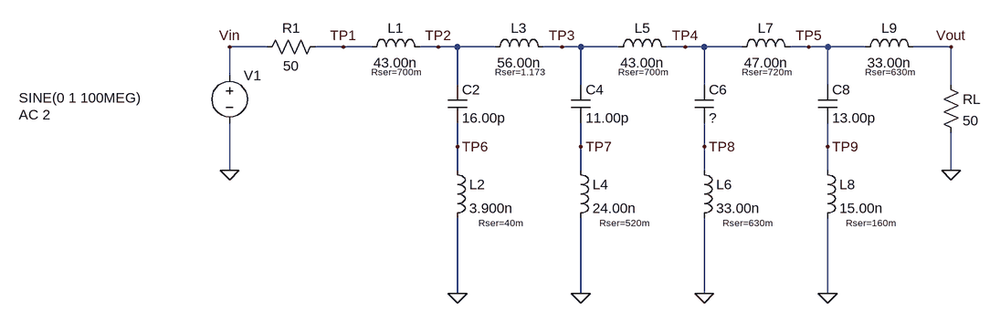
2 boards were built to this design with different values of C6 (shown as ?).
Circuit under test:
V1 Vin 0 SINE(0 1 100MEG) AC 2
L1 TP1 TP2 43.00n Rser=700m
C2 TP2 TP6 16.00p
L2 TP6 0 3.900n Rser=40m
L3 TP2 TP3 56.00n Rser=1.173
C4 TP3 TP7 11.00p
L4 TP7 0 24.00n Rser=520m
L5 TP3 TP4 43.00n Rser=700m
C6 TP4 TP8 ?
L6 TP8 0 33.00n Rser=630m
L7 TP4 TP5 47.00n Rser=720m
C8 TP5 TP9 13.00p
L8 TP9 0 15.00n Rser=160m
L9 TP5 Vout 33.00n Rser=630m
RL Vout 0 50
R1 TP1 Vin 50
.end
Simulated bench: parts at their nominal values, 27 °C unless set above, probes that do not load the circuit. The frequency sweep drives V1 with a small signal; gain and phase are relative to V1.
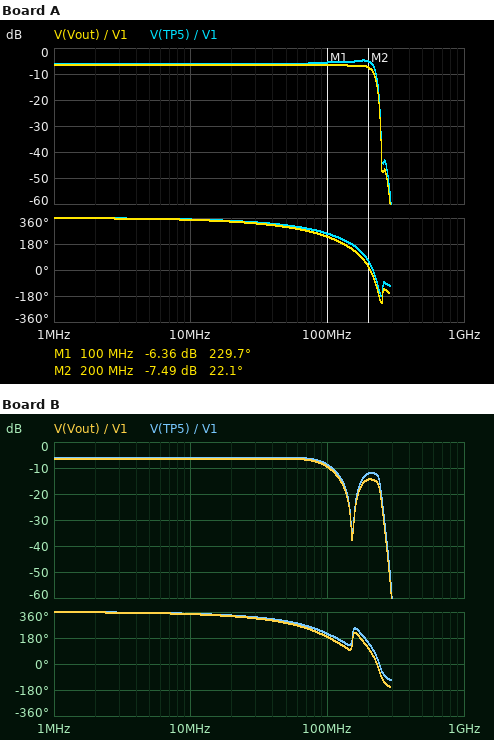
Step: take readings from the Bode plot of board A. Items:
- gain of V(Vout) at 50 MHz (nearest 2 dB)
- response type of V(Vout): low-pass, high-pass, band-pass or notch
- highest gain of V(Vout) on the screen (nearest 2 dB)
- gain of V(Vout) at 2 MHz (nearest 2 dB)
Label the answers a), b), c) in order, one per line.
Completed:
a) -6 dB
b) low-pass
c) -6 dB
d) -6 dB
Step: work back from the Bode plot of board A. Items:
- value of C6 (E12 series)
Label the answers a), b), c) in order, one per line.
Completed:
a) 12 pF
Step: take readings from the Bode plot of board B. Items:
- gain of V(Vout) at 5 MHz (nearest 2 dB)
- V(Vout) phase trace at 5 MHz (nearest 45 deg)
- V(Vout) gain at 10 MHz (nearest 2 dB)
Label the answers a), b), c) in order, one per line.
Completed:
a) -6 dB
b) 360 deg
c) -6 dB
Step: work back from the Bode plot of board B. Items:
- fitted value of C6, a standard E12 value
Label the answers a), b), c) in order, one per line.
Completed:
a) 33 pF
